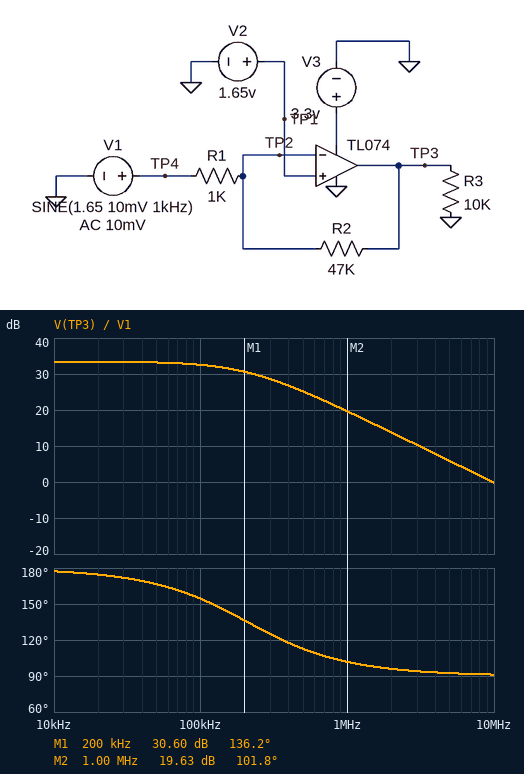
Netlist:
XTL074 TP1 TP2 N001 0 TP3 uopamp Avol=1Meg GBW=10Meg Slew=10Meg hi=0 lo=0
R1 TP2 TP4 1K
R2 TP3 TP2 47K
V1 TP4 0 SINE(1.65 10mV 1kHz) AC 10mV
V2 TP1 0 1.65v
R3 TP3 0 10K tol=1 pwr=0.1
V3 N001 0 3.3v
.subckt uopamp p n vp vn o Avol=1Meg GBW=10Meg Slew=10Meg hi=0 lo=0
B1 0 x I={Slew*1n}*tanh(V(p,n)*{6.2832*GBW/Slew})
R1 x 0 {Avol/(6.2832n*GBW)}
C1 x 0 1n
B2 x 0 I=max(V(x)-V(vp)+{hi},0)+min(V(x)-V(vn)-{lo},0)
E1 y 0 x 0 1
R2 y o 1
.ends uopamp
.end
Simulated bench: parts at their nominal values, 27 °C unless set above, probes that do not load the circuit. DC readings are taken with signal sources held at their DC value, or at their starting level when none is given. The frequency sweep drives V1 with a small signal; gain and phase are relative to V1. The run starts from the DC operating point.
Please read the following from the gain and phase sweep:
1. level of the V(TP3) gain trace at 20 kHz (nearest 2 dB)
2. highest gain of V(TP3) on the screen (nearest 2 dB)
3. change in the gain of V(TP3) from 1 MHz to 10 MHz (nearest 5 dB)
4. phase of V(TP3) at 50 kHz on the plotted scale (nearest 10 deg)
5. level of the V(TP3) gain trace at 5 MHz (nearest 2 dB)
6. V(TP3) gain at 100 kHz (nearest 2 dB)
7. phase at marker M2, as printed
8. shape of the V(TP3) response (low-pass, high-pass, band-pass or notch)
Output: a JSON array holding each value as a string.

["34 dB", "34 dB", "-20 dB", "170 deg", "6 dB", "32 dB", "101.8 deg", "low-pass"]
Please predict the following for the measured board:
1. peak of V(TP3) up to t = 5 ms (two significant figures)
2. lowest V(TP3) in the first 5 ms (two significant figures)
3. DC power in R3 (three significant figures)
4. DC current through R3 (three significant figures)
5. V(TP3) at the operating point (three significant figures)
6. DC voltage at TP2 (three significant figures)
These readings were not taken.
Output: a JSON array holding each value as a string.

["2.1 V", "1.2 V", "272 µW", "165 µA", "1.65 V", "1.65 V"]
